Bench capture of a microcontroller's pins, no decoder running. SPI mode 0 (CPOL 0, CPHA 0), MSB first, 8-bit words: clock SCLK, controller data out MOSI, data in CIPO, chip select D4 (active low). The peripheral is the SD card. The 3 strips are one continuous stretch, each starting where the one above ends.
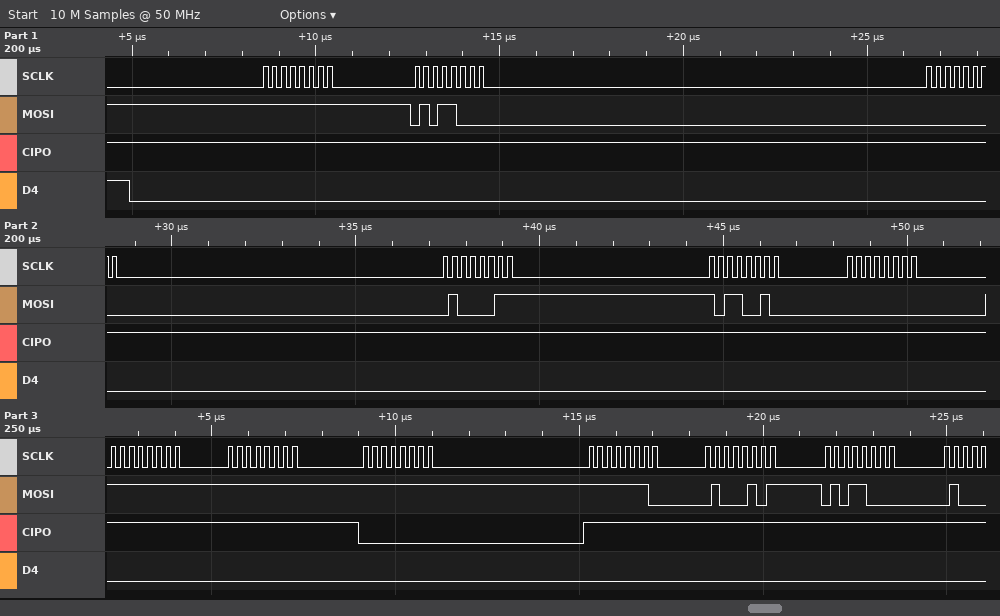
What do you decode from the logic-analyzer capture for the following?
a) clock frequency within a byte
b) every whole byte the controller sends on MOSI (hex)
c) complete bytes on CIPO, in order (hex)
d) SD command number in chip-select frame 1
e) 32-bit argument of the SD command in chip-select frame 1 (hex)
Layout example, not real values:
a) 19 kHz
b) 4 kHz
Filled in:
a) 4 MHz
b) FF 58 00 43 B2 00 FF FF FF FE 45 58
c) FF FF FF FF FF FF FF FF 00 FF FF FF
d) CMD24
e) 0x0043B200
